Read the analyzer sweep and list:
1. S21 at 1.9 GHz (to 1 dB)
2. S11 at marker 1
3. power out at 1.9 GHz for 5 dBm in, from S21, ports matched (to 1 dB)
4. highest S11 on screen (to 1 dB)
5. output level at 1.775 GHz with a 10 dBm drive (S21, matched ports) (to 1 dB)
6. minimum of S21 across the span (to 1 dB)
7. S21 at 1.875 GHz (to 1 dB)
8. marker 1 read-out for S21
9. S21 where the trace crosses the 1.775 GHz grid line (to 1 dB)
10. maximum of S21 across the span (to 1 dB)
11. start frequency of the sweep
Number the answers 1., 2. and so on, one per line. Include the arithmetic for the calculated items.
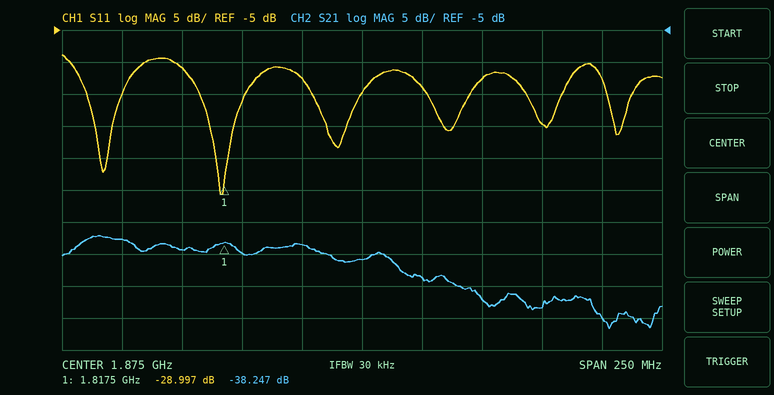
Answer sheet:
1. -44 dB
2. -28.997 dB
3. 5 dBm + (-44 dB) = -39 dBm
4. -9 dB
5. 10 dBm + (-38 dB) = -28 dBm
6. -52 dB
7. -41 dB
8. -38.247 dB
9. -38 dB
10. -37 dB
11. 1.75 GHz
